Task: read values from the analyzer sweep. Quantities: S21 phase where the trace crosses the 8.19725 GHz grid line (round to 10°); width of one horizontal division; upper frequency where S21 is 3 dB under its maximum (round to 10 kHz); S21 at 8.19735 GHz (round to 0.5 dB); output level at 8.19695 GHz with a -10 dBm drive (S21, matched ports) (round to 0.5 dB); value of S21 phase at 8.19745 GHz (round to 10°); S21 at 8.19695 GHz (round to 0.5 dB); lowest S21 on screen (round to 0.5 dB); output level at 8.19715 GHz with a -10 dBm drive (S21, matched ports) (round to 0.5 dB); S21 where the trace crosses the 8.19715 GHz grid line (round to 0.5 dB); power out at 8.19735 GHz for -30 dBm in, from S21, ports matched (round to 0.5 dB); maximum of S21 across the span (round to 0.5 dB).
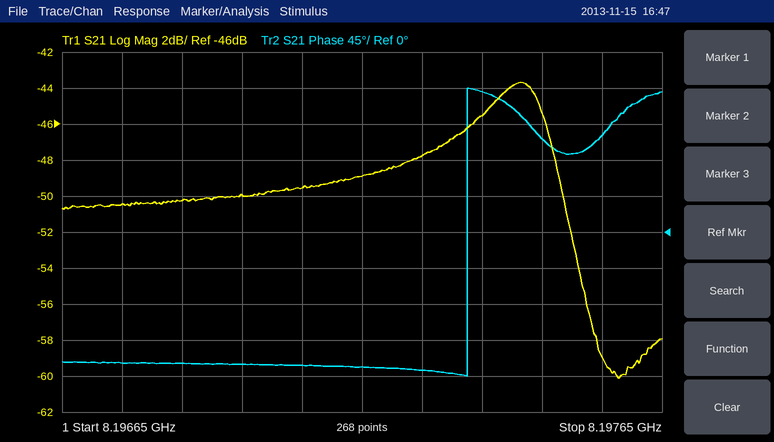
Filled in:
-170°
100 kHz
8.19746 GHz
-45.5 dB
-60.0 dBm
120°
-50.0 dB
-60.0 dB
-59.0 dBm
-49.0 dB
-75.5 dBm
-43.5 dB
